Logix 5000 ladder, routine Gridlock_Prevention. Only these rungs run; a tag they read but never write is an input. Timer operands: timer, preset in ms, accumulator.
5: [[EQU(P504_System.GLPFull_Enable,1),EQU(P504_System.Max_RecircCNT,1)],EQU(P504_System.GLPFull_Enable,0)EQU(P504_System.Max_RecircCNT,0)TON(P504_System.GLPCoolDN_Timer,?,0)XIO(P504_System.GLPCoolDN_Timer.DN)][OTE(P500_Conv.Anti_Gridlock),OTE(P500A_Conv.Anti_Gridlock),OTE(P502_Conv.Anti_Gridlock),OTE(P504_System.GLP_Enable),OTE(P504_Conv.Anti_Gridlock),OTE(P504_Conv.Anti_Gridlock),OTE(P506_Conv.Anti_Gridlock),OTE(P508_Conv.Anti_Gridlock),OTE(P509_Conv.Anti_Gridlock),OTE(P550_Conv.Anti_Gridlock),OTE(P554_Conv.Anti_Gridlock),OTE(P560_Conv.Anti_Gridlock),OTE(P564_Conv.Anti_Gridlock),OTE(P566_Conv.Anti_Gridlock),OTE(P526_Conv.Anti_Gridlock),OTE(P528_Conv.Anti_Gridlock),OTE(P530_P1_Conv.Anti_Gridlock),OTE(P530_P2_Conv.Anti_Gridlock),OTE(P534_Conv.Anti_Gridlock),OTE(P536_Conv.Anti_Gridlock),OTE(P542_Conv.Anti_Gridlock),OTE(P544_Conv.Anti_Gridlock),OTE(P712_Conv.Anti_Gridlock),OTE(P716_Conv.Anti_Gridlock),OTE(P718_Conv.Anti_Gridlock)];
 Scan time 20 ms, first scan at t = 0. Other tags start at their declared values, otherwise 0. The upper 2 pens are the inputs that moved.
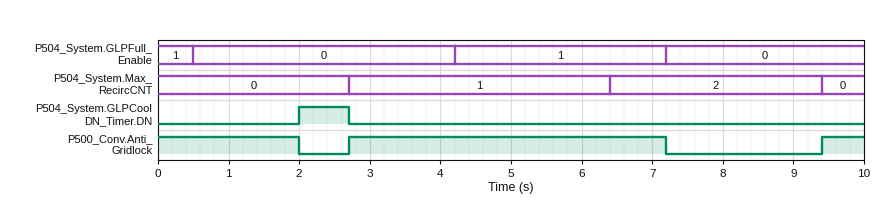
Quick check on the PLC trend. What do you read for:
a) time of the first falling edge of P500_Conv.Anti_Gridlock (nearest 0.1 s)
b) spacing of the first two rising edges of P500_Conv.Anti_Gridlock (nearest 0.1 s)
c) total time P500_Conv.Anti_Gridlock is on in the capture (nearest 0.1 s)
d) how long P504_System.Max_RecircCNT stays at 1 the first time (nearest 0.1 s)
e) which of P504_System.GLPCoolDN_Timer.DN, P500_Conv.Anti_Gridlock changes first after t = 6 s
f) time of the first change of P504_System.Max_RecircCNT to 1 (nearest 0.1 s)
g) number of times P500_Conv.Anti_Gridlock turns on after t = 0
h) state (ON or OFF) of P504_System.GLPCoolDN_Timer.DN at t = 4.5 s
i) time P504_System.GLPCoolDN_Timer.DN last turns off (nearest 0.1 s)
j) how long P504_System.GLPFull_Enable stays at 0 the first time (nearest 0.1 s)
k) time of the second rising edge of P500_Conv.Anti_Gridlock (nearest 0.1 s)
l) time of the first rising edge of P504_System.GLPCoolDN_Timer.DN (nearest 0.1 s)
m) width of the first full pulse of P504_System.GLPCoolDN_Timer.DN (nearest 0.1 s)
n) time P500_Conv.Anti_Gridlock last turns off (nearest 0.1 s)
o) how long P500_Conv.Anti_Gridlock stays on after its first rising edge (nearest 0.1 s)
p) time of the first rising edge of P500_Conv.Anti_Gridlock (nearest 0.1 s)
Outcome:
2.0 s
6.7 s
7.1 s
3.7 s
P500_Conv.Anti_Gridlock
2.7 s
2
OFF
2.7 s
3.7 s
9.4 s
2.0 s
0.7 s
7.2 s
4.5 s
2.7 s
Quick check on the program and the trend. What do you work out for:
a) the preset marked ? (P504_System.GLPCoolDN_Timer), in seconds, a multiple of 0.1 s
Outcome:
1.5 s
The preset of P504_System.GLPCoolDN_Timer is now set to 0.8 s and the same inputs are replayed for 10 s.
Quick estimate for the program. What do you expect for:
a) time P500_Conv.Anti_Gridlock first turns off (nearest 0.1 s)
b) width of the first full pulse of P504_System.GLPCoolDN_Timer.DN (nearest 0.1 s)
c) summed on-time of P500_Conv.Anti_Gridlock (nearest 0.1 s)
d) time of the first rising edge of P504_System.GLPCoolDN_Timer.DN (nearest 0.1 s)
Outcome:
1.3 s
1.4 s
6.4 s
1.3 s
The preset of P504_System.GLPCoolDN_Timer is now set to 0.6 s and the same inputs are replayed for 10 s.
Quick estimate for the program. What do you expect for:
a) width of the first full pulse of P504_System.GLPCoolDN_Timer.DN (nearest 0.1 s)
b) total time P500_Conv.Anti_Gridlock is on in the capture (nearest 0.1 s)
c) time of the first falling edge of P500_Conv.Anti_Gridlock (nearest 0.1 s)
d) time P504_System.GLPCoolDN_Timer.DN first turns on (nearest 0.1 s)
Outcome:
1.6 s
6.2 s
1.1 s
1.1 s
